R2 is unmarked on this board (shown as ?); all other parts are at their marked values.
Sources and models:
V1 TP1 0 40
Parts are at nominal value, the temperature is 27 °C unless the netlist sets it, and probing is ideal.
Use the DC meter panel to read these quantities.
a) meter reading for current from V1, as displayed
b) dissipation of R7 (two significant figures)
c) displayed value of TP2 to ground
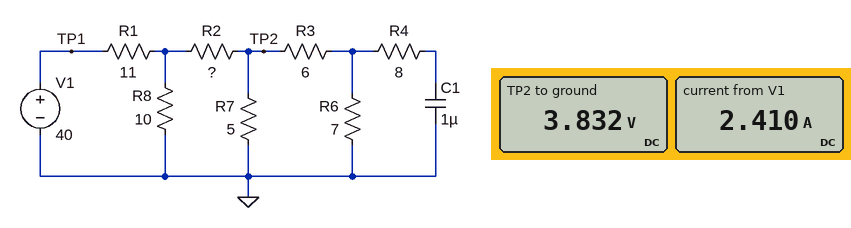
2.410 A
2.9 W
3.832 V
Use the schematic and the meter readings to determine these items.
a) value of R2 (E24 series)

9.1 Ω
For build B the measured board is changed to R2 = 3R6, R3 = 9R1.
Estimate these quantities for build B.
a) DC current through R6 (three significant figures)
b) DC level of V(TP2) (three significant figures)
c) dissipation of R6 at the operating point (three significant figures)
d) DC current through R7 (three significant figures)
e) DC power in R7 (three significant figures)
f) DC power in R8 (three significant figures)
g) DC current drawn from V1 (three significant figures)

357 mA
5.74 V
891 mW
1.15 A
6.60 W
12.5 W
2.62 A
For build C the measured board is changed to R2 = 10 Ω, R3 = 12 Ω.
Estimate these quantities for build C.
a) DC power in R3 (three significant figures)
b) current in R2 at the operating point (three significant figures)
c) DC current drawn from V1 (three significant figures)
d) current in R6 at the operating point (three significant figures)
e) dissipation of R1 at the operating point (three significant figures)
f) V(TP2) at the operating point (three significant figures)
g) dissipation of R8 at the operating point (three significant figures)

513 mW
992 mA
2.38 A
207 mA
62.2 W
3.93 V
19.2 W
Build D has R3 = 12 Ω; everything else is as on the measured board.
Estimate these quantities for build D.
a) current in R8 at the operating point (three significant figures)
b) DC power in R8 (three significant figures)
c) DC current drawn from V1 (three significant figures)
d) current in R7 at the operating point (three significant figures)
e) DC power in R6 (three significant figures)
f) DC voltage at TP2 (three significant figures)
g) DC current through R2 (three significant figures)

1.36 A
18.5 W
2.40 A
824 mA
329 mW
4.12 V
1.04 A
